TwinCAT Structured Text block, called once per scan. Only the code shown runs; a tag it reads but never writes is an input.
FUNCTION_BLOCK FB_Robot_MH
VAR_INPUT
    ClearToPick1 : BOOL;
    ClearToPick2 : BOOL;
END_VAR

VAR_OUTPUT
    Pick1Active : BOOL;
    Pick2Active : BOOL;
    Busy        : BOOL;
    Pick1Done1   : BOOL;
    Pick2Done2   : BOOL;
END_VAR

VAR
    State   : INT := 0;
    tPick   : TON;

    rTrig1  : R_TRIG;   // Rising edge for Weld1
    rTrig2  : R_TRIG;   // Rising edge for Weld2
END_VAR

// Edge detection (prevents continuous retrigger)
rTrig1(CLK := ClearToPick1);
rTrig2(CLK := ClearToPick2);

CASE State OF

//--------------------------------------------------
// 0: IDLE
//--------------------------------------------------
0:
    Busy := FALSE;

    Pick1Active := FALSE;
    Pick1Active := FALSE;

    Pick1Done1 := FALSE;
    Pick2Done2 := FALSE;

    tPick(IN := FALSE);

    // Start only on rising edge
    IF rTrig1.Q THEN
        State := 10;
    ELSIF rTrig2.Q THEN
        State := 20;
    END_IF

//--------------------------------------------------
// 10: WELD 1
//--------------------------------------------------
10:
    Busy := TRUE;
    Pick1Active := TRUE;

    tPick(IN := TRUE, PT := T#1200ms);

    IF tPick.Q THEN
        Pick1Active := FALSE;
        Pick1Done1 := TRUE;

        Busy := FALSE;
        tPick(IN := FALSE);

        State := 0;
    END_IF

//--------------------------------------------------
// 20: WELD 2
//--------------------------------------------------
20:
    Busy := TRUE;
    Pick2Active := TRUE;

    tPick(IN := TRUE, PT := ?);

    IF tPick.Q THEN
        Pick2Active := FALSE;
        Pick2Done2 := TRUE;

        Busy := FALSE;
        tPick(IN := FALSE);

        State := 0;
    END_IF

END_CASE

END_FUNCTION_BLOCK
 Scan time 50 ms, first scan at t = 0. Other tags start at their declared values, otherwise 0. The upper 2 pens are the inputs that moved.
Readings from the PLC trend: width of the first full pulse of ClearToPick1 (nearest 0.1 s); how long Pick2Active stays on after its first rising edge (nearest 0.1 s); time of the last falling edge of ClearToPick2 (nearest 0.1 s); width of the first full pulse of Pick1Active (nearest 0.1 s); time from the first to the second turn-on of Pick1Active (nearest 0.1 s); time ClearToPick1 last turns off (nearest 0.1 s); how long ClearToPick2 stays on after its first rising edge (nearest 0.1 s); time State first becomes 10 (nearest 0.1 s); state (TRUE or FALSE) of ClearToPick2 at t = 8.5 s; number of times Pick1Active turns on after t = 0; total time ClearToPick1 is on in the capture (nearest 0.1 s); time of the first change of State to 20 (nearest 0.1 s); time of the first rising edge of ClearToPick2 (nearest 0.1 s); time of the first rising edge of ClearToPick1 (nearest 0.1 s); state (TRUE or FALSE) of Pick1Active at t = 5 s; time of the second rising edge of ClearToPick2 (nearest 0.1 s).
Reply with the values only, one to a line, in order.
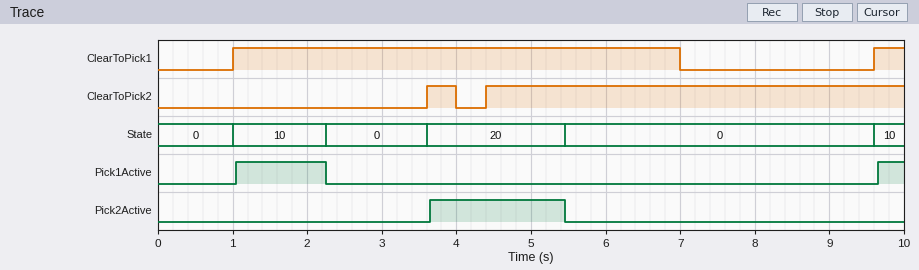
6.0 s
1.8 s
4.0 s
1.2 s
8.6 s
7.0 s
0.4 s
1.0 s
TRUE
2
6.4 s
3.6 s
3.6 s
1.0 s
FALSE
4.4 s
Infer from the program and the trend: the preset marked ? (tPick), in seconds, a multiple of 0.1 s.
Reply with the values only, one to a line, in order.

1.8 s
